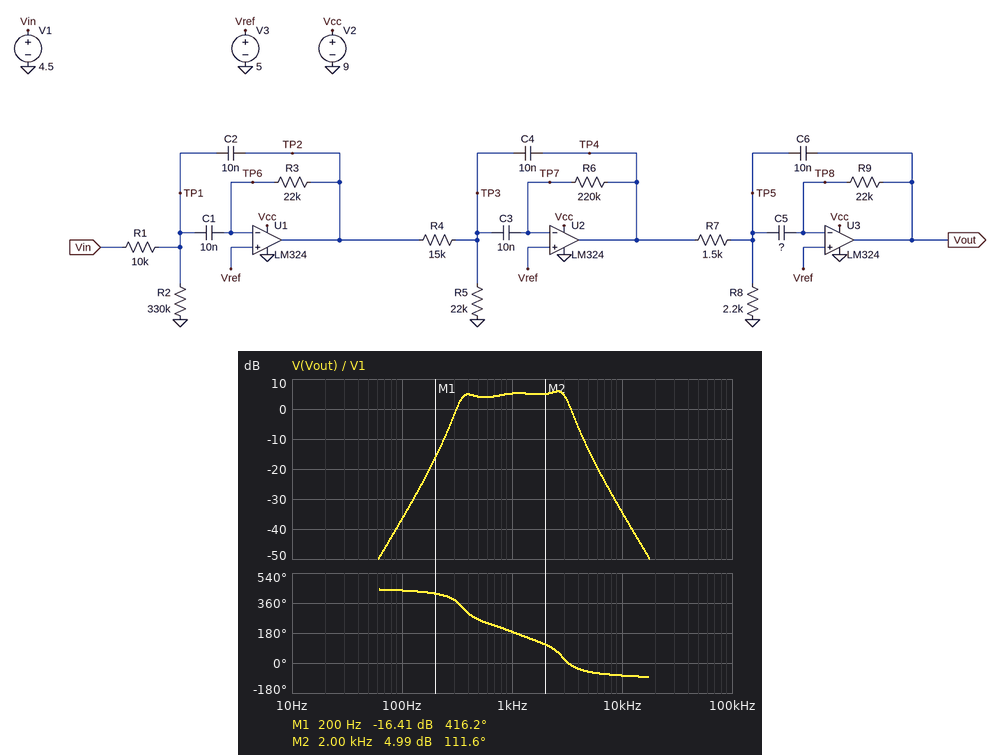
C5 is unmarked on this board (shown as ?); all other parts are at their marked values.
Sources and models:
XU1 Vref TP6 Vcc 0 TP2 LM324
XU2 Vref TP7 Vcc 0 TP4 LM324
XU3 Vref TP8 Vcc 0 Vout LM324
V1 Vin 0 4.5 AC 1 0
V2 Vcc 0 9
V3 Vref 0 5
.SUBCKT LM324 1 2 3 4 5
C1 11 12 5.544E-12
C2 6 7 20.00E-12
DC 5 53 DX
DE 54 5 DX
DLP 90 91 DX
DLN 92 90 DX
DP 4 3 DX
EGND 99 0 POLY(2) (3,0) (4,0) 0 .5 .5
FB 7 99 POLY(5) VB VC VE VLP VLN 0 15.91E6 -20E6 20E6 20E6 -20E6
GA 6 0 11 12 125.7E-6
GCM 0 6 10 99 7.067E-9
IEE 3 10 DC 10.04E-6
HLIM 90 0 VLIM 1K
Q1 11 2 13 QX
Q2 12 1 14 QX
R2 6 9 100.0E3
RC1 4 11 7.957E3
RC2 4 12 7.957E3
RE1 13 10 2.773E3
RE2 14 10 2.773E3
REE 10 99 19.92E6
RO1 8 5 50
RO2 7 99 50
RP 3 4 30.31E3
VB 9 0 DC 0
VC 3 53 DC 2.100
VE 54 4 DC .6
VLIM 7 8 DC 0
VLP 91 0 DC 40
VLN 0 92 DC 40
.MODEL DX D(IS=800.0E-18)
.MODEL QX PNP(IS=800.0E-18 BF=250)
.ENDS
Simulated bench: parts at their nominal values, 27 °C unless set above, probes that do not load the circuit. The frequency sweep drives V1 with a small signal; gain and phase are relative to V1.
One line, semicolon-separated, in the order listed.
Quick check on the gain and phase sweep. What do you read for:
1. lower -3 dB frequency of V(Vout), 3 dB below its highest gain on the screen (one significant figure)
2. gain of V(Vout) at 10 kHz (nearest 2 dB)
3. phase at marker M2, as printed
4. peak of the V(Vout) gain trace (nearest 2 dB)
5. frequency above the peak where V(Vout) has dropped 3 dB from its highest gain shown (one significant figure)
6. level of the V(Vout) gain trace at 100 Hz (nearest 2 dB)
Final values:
300 Hz; -34 dB; 111.6 deg; 6 dB; 3 kHz; -36 dB
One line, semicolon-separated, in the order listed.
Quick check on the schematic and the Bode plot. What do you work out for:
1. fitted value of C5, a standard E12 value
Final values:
15 nF
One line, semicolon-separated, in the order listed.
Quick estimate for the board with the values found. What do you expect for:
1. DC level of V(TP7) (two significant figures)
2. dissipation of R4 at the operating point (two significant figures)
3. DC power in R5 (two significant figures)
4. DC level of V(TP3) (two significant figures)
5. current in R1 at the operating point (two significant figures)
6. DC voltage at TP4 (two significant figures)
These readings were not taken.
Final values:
5.0 V; 270 µW; 400 µW; 3.0 V; 13 µA; 5.0 V
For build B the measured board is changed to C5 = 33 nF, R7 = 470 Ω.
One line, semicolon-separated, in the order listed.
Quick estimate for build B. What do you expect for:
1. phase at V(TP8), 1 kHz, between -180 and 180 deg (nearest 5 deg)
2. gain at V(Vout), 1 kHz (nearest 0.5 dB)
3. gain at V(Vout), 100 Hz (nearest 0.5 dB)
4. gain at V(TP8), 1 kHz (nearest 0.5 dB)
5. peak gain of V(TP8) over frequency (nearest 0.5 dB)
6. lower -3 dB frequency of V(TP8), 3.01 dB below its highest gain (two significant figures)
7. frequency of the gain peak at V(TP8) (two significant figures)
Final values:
100 deg; 15.0 dB; -27.0 dB; -45.0 dB; -33.5 dB; 2.4 kHz; 2.9 kHz
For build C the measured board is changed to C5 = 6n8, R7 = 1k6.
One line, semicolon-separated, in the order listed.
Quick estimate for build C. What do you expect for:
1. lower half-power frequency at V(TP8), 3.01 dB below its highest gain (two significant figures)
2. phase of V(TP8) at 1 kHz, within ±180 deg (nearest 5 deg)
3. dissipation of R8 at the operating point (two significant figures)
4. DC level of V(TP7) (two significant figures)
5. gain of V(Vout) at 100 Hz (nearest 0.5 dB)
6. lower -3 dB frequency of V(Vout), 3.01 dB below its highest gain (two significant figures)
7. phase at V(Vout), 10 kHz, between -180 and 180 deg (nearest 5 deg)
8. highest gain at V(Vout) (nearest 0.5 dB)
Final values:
3.0 kHz; 100 deg; 3.8 mW; 5.0 V; -44.0 dB; 330 Hz; -70 deg; -2.5 dB
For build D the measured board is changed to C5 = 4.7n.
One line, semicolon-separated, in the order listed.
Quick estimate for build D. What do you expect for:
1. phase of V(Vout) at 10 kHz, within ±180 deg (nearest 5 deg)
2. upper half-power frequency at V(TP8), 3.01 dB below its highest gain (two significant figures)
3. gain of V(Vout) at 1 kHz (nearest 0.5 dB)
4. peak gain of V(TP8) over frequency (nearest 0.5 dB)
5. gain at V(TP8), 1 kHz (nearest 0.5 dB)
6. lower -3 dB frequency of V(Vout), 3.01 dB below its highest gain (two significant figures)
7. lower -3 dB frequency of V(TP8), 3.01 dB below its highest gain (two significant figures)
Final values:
-65 deg; 6.0 kHz; -5.5 dB; -56.0 dB; -65.5 dB; 330 Hz; 3.6 kHz
